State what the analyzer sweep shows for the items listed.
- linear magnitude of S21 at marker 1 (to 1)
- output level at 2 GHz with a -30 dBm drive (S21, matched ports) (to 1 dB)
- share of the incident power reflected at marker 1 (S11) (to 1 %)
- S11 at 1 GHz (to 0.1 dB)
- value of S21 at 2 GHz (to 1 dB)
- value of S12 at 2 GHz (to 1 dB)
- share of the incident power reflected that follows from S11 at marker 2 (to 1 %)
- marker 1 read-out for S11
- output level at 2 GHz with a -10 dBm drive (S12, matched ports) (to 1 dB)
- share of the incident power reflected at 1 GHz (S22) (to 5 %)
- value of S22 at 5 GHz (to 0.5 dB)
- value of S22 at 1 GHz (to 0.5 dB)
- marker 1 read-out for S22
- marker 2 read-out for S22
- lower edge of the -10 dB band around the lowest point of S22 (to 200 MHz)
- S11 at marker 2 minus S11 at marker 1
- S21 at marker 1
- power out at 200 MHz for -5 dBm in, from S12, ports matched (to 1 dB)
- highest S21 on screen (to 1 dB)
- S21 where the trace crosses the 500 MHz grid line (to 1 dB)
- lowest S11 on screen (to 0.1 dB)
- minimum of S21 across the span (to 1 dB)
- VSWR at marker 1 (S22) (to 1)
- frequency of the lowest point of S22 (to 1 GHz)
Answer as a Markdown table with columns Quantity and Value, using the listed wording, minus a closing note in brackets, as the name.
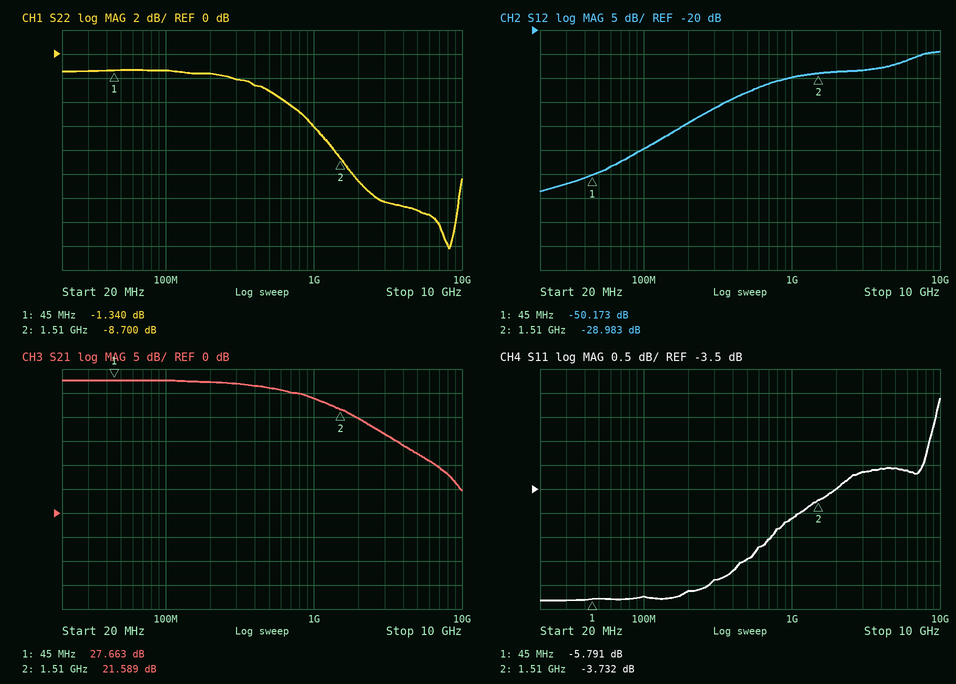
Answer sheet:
| Quantity | Value |
|---|---|
| linear magnitude of S21 at marker 1 | 24 |
| output level at 2 GHz with a -30 dBm drive (S21, matched ports) | -10 dBm |
| share of the incident power reflected at marker 1 (S11) | 26 % |
| S11 at 1 GHz | -4.1 dB |
| value of S21 at 2 GHz | 20 dB |
| value of S12 at 2 GHz | -29 dB |
| share of the incident power reflected that follows from S11 at marker 2 | 42 % |
| marker 1 read-out for S11 | -5.791 dB |
| output level at 2 GHz with a -10 dBm drive (S12, matched ports) | -39 dBm |
| share of the incident power reflected at 1 GHz (S22) | 25 % |
| value of S22 at 5 GHz | -13.0 dB |
| value of S22 at 1 GHz | -6.0 dB |
| marker 1 read-out for S22 | -1.340 dB |
| marker 2 read-out for S22 | -8.700 dB |
| lower edge of the -10 dB band around the lowest point of S22 | 1.8 GHz |
| S11 at marker 2 minus S11 at marker 1 | 2.059 dB |
| S21 at marker 1 | 27.663 dB |
| power out at 200 MHz for -5 dBm in, from S12, ports matched | -44 dBm |
| highest S21 on screen | 28 dB |
| S21 where the trace crosses the 500 MHz grid line | 26 dB |
| lowest S11 on screen | -5.8 dB |
| minimum of S21 across the span | 5 dB |
| VSWR at marker 1 (S22) | 13 |
| frequency of the lowest point of S22 | 8 GHz |
